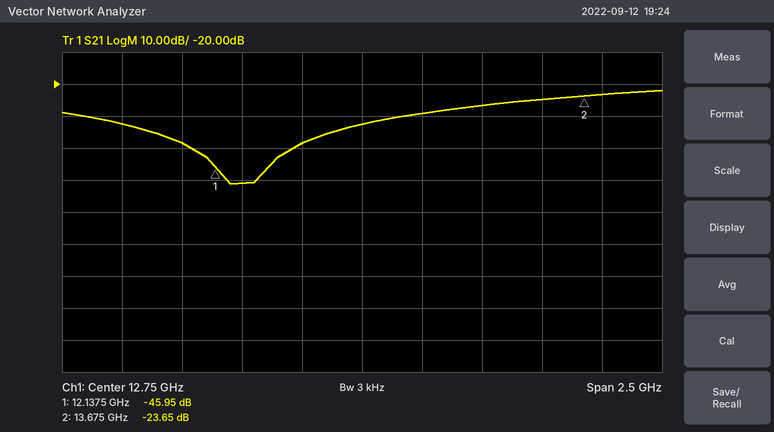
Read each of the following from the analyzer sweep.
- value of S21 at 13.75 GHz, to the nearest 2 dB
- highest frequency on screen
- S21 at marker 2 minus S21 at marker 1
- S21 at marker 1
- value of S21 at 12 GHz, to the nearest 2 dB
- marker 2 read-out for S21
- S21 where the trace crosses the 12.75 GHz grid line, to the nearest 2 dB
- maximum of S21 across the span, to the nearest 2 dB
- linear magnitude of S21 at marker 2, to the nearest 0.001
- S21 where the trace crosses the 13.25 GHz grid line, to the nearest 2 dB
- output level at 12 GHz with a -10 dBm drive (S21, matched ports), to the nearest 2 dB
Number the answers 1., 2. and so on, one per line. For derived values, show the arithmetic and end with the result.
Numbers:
1. -24 dB
2. 14 GHz
3. -23.65 − (-45.95) = 22.30 dB
4. -45.95 dB
5. -38 dB
6. -23.65 dB
7. -32 dB
8. -22 dB
9. 10^(-23.65/20) ≈ 0.066
10. -26 dB
11. -10 dBm + (-38 dB) = -48 dBm
